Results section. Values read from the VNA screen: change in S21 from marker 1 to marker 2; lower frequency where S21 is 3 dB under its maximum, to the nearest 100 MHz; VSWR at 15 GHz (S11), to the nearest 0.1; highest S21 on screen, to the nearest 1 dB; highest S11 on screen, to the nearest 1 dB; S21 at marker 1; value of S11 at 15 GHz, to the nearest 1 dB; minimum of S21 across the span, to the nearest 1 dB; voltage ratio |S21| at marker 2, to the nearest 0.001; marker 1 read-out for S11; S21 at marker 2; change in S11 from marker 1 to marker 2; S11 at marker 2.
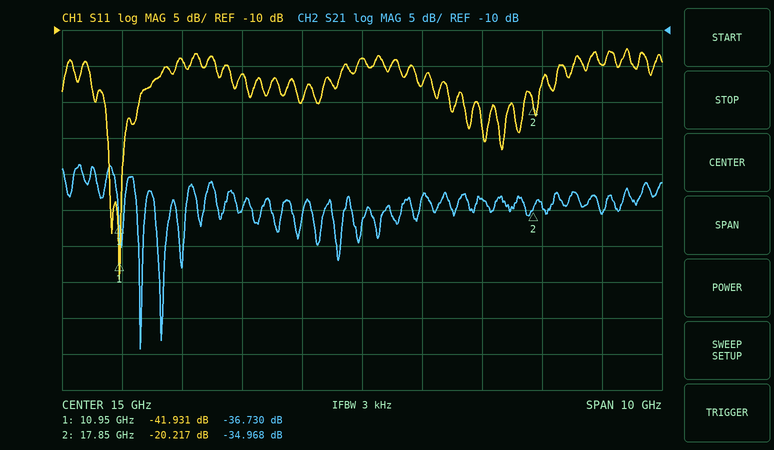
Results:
1.762 dB
10.2 GHz
1.5
-29 dB
-13 dB
-36.730 dB
-14 dB
-54 dB
0.018
-41.931 dB
-34.968 dB
21.714 dB
-20.217 dB
